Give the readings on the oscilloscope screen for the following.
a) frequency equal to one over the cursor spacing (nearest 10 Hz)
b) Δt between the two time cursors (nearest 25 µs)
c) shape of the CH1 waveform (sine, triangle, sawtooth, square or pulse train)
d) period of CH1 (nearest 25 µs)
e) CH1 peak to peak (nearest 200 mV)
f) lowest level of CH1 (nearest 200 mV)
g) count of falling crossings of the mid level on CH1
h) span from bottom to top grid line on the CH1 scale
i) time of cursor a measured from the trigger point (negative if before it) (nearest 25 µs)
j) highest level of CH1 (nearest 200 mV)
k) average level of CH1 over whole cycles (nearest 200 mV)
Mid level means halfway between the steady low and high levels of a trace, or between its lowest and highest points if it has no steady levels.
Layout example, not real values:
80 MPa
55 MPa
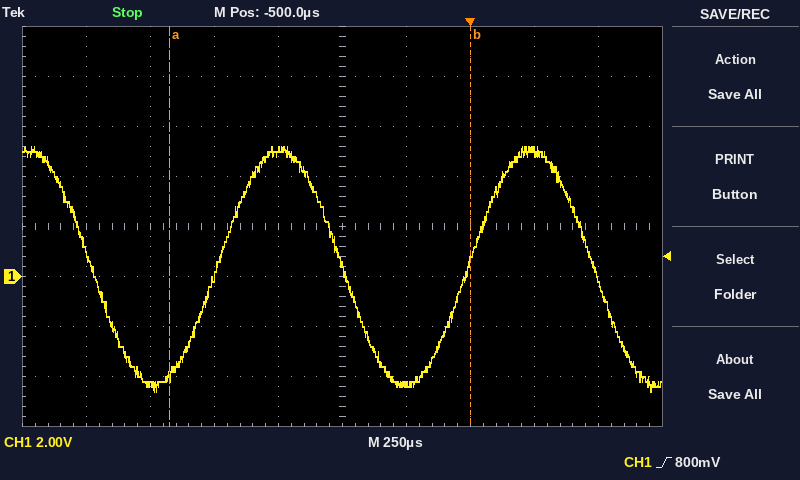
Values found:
850 Hz
1.175 ms
sine
975 µs
9.8 V
-4.6 V
3
16 V
-1.175 ms
5.2 V
400 mV
